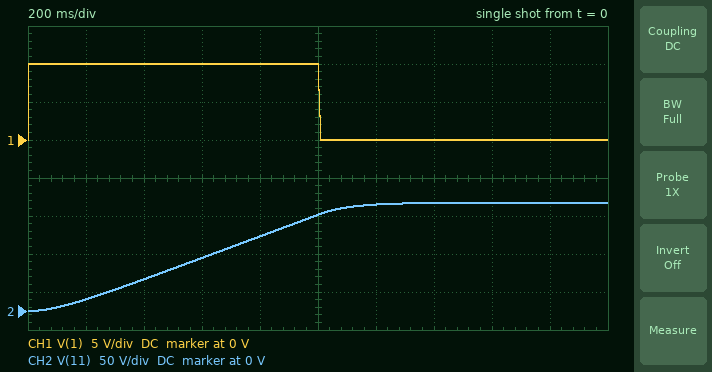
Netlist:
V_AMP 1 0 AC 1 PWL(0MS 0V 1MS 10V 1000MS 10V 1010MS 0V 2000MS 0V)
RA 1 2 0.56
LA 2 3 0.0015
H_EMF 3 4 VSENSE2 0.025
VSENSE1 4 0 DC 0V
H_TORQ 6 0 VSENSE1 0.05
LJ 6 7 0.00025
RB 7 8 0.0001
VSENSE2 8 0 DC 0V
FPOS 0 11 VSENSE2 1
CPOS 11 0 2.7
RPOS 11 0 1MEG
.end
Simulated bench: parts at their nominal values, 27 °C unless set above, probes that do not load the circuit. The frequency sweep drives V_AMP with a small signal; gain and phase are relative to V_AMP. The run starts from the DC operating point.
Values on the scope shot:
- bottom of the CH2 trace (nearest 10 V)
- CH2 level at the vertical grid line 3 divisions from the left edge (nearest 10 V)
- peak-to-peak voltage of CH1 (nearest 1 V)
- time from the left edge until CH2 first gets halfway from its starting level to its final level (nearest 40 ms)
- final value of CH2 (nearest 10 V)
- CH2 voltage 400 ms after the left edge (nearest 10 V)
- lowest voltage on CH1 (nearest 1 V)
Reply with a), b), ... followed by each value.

a) 0 V
b) 70 V
c) 10 V
d) 600 ms
e) 140 V
f) 40 V
g) 0 V
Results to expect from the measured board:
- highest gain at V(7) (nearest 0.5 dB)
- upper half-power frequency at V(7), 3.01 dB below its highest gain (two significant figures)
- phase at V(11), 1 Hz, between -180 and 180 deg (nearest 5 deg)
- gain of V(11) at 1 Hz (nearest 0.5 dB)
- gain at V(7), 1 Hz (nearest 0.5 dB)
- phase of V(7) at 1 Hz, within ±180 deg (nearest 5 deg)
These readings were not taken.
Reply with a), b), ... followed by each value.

a) -48.5 dB
b) 1.5 Hz
c) -125 deg
d) 5.5 dB
e) -50.0 dB
f) -35 deg
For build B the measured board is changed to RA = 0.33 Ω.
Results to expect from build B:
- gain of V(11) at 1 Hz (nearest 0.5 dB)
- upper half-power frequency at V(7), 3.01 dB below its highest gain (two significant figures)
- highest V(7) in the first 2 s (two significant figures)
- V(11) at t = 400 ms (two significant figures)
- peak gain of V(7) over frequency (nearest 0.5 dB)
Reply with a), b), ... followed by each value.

a) 6.5 dB
b) 2.7 Hz
c) 39 mV
d) 48 V
e) -48.0 dB
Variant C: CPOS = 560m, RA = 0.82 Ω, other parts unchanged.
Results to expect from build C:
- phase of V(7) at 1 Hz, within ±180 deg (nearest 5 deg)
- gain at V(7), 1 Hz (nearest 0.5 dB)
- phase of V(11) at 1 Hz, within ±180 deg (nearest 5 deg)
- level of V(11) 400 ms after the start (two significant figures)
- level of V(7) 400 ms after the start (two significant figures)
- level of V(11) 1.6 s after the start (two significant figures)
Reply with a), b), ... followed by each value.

a) -45 deg
b) -51.5 dB
c) -135 deg
d) 170 V
e) 35 mV
f) 670 V
